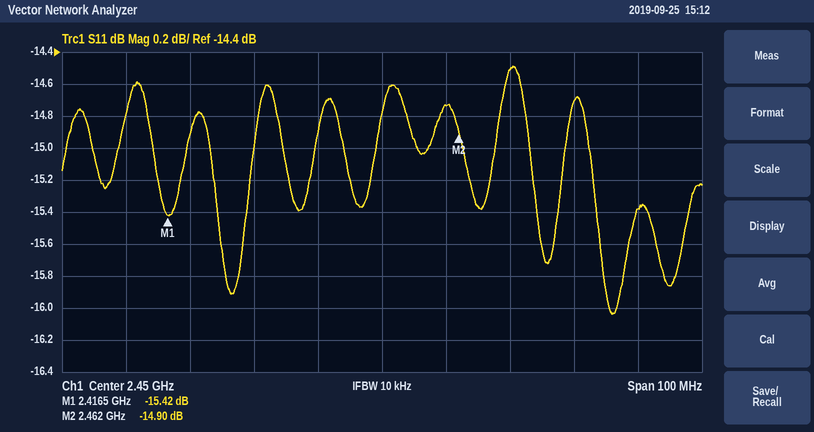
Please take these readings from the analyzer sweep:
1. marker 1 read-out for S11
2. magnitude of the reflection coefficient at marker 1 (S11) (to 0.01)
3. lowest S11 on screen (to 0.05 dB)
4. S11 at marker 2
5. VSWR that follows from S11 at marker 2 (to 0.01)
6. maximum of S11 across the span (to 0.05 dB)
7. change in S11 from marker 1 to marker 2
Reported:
-15.42 dB
0.17
-16.05 dB
-14.90 dB
1.44
-14.50 dB
0.52 dB
